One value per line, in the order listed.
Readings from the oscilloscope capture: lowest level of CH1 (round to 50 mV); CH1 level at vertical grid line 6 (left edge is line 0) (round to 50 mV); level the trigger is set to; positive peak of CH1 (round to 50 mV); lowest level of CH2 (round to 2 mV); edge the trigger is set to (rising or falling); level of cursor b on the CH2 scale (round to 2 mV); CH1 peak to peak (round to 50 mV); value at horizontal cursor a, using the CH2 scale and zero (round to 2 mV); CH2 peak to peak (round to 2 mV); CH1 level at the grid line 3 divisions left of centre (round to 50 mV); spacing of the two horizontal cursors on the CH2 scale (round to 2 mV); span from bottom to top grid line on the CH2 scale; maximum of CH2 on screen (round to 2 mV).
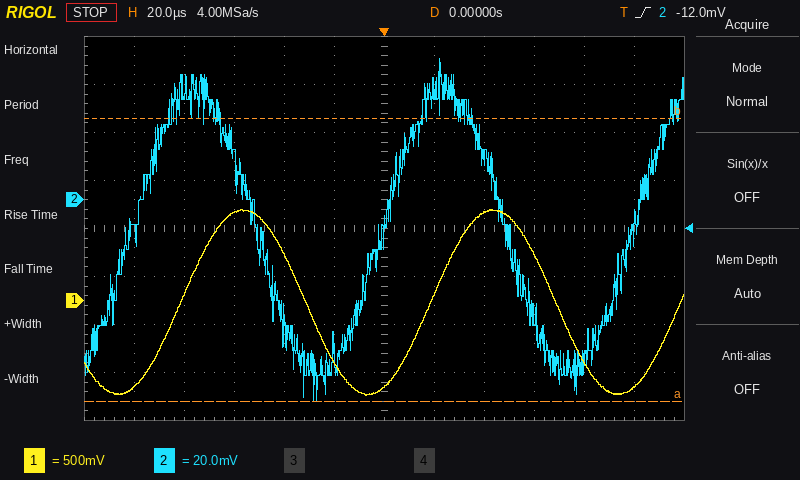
-1.00 V
-900 mV
-12.0 mV
950 mV
-84 mV
rising
34 mV
1.95 V
-84 mV
142 mV
900 mV
118 mV
160 mV
58 mV
